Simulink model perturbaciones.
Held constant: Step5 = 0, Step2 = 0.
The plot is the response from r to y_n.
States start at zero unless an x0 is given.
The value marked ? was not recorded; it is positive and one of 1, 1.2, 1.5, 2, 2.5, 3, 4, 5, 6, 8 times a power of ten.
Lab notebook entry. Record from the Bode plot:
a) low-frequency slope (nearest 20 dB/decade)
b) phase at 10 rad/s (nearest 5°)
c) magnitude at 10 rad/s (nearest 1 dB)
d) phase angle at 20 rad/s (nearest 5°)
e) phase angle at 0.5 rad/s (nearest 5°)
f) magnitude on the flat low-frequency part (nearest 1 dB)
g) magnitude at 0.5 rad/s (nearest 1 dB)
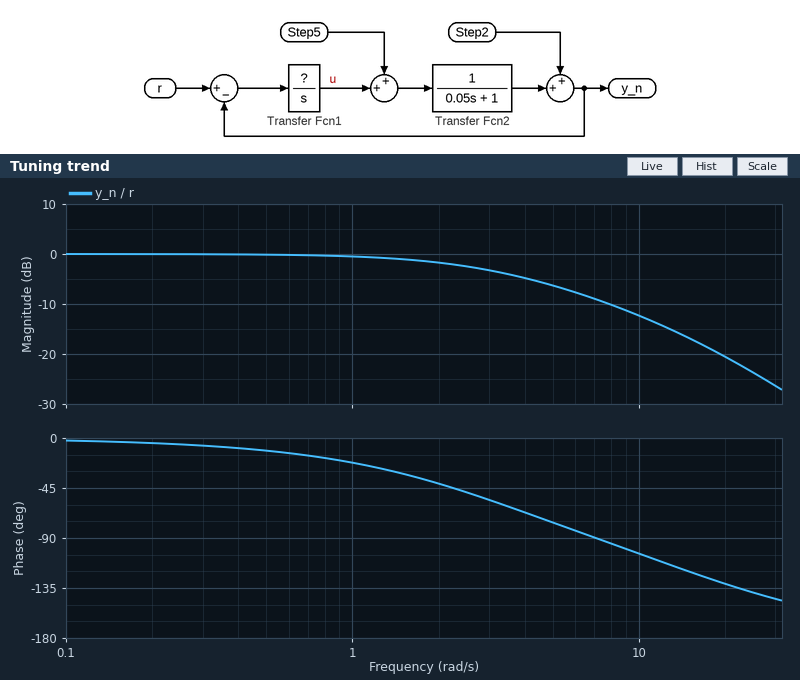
0 dB/decade
-105°
-12 dB
-130°
-10°
0 dB
0 dB
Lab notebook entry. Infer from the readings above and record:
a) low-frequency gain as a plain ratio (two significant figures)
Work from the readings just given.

1.0
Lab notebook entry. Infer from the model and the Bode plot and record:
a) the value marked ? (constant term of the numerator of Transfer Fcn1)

2.5
